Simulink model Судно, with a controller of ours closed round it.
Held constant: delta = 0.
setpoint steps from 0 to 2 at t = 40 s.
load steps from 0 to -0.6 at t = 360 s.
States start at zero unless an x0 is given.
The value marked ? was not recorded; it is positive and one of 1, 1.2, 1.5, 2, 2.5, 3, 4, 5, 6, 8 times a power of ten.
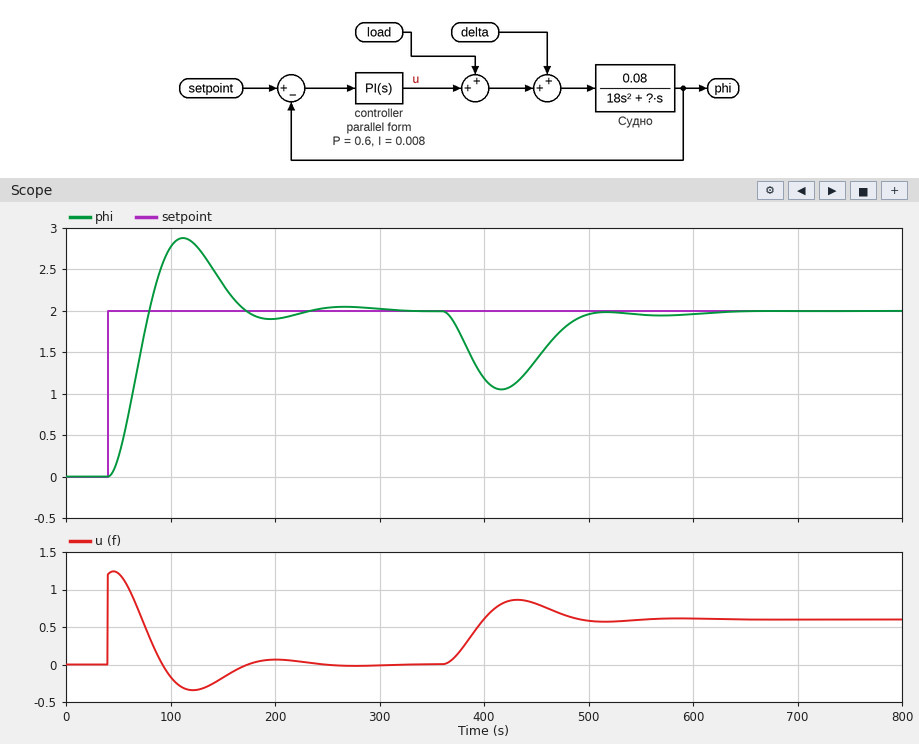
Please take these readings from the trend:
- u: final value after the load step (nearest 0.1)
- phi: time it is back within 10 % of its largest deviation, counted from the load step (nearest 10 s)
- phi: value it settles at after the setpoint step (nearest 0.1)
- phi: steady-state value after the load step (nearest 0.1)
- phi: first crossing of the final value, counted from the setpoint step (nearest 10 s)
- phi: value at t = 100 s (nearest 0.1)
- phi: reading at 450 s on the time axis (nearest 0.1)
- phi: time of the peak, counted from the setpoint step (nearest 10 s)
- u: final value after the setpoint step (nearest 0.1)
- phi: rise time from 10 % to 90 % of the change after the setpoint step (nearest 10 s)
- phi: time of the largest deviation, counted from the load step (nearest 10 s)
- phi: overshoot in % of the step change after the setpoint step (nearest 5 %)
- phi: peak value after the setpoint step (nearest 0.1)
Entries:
0.6
130 s
2.0
2.0
40 s
2.8
1.4
70 s
0.0
30 s
60 s
45 %
2.9
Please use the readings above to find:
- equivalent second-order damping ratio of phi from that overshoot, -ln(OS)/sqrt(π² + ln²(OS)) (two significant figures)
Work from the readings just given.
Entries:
0.25
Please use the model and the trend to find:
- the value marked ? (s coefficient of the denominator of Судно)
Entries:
1
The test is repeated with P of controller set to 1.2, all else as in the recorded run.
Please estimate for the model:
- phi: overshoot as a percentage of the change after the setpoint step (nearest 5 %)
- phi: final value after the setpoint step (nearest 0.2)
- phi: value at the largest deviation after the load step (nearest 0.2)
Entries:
40 %
2.0
1.4
